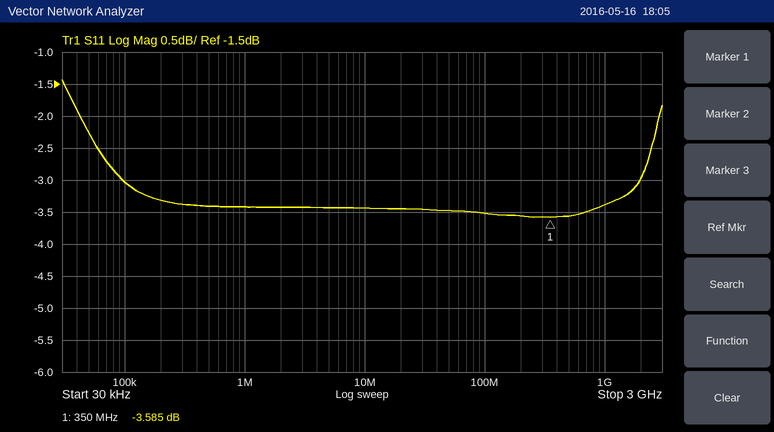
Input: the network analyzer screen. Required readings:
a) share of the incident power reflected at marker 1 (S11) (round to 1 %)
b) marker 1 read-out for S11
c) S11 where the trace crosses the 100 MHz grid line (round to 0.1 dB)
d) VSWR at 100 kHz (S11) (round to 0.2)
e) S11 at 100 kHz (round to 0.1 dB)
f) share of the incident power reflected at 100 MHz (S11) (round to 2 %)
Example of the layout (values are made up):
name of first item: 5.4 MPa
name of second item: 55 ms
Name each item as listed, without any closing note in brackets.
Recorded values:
share of the incident power reflected at marker 1 (S11): 44 %
marker 1 read-out for S11: -3.585 dB
S11 where the trace crosses the 100 MHz grid line: -3.5 dB
VSWR at 100 kHz (S11): 5.8
S11 at 100 kHz: -3.0 dB
share of the incident power reflected at 100 MHz (S11): 44 %
